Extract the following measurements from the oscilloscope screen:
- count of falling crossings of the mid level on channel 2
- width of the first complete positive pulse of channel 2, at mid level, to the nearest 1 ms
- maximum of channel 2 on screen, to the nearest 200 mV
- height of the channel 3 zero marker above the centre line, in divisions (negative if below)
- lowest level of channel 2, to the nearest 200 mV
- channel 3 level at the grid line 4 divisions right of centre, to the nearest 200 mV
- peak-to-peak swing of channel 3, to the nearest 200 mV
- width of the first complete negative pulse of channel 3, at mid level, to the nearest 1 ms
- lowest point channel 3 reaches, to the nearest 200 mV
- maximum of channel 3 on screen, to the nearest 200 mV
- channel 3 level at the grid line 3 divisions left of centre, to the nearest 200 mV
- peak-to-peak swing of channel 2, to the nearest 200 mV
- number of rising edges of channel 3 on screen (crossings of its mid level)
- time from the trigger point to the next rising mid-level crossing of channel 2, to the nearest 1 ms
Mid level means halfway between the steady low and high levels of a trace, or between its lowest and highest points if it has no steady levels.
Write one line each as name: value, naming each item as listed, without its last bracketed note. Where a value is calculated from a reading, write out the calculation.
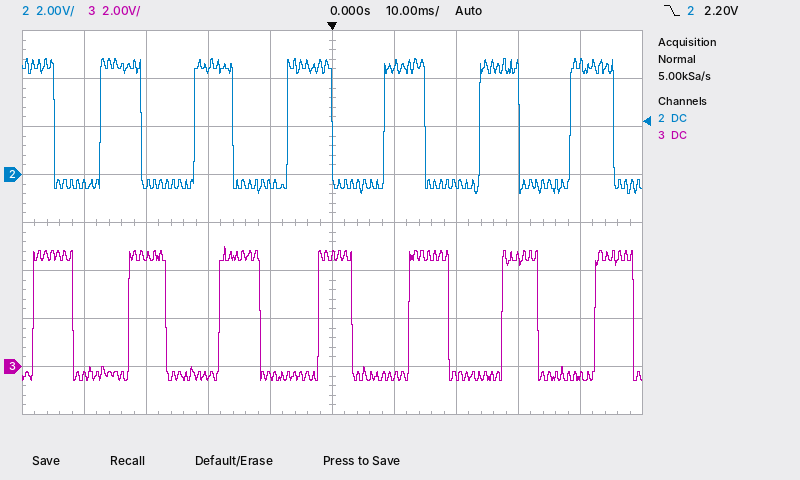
count of falling crossings of the mid level on channel 2: 7
width of the first complete positive pulse of channel 2, at mid level, to the nearest 1 ms: 7 ms
maximum of channel 2 on screen, to the nearest 200 mV: 4.8 V
height of the channel 3 zero marker above the centre line, in divisions: -3.0 div
lowest level of channel 2, to the nearest 200 mV: -800 mV
channel 3 level at the grid line 4 divisions right of centre, to the nearest 200 mV: -400 mV
peak-to-peak swing of channel 3, to the nearest 200 mV: 5.0 V − (-600 mV) = 5.6 V
width of the first complete negative pulse of channel 3, at mid level, to the nearest 1 ms: 9 ms
lowest point channel 3 reaches, to the nearest 200 mV: -600 mV
maximum of channel 3 on screen, to the nearest 200 mV: 5.0 V
channel 3 level at the grid line 3 divisions left of centre, to the nearest 200 mV: 4.6 V
peak-to-peak swing of channel 2, to the nearest 200 mV: 4.8 V − (-800 mV) = 5.6 V
number of rising edges of channel 3 on screen: 7
time from the trigger point to the next rising mid-level crossing of channel 2, to the nearest 1 ms: 8 ms
